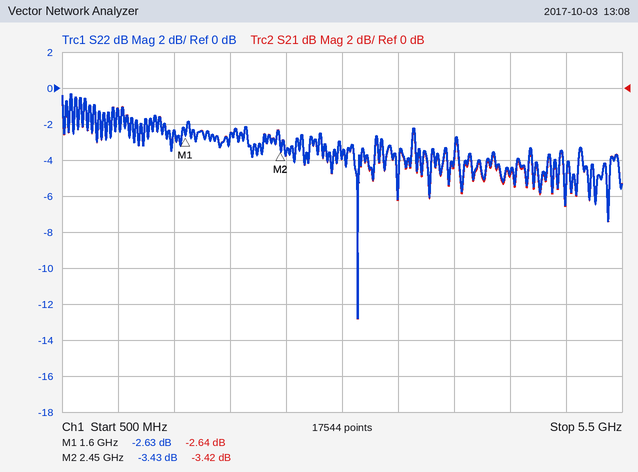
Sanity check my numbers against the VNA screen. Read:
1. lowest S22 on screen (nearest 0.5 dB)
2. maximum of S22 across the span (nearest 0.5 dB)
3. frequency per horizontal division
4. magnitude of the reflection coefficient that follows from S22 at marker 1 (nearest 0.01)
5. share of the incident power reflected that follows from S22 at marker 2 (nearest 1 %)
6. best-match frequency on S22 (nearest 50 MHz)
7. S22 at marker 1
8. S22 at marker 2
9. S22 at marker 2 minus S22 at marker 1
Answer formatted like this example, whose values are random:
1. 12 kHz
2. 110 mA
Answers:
1. -13.0 dB
2. -0.5 dB
3. 500 MHz
4. 0.74
5. 45 %
6. 3.15 GHz
7. -2.63 dB
8. -3.43 dB
9. -0.80 dB
